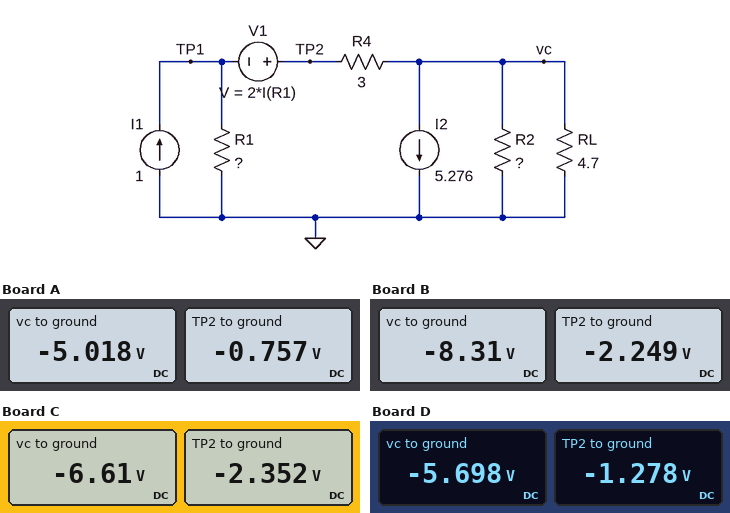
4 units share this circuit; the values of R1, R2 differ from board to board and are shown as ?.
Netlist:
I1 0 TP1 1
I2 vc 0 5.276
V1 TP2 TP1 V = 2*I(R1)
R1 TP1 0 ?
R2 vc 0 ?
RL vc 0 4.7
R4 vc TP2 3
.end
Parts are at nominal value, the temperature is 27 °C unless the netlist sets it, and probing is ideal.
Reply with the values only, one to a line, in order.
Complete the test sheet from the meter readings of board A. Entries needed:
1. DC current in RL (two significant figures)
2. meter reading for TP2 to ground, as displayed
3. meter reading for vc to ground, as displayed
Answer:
1.1 A
-0.757 V
-5.018 V
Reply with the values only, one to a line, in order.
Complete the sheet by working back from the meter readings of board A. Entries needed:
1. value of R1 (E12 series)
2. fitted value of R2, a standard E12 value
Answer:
1.8 Ω
1.8 Ω
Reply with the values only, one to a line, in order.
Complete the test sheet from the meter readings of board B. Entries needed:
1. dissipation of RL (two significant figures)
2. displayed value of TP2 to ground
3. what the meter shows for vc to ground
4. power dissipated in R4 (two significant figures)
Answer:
15 W
-2.249 V
-8.31 V
12 W
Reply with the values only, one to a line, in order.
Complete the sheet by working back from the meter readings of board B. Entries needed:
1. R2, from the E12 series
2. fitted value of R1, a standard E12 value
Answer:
5.6 Ω
2.2 Ω
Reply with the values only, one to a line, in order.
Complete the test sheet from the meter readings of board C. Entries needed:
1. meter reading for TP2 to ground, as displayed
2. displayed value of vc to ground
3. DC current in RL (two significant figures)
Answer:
-2.352 V
-6.61 V
1.4 A
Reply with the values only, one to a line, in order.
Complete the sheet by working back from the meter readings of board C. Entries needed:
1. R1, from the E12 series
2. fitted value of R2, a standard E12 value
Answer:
5.6 Ω
2.7 Ω
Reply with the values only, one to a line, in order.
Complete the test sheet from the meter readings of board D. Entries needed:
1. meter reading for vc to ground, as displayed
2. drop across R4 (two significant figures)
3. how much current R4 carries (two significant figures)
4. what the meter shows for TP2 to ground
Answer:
-5.698 V
4.4 V
1.5 A
-1.278 V
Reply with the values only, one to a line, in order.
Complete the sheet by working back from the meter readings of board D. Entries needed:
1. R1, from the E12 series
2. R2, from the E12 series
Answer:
2.7 Ω
2.2 Ω
